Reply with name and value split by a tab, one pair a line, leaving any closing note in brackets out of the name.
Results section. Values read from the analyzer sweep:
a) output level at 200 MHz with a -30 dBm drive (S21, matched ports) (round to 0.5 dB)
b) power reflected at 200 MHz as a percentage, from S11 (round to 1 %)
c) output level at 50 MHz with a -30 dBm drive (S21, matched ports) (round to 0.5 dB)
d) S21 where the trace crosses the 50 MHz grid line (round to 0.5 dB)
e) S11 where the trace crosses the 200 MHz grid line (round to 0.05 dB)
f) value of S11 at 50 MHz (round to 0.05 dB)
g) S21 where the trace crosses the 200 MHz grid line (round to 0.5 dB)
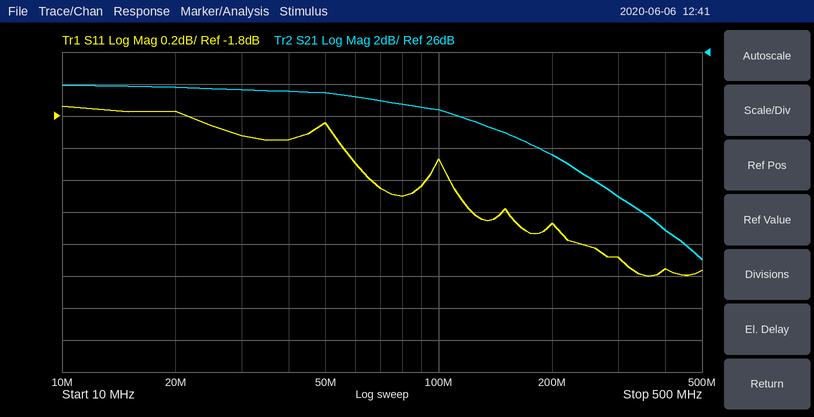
output level at 200 MHz with a -30 dBm drive (S21, matched ports)	-10.5 dBm
power reflected at 200 MHz as a percentage, from S11	57 %
output level at 50 MHz with a -30 dBm drive (S21, matched ports)	-6.5 dBm
S21 where the trace crosses the 50 MHz grid line	23.5 dB
S11 where the trace crosses the 200 MHz grid line	-2.45 dB
value of S11 at 50 MHz	-1.85 dB
S21 where the trace crosses the 200 MHz grid line	19.5 dB
